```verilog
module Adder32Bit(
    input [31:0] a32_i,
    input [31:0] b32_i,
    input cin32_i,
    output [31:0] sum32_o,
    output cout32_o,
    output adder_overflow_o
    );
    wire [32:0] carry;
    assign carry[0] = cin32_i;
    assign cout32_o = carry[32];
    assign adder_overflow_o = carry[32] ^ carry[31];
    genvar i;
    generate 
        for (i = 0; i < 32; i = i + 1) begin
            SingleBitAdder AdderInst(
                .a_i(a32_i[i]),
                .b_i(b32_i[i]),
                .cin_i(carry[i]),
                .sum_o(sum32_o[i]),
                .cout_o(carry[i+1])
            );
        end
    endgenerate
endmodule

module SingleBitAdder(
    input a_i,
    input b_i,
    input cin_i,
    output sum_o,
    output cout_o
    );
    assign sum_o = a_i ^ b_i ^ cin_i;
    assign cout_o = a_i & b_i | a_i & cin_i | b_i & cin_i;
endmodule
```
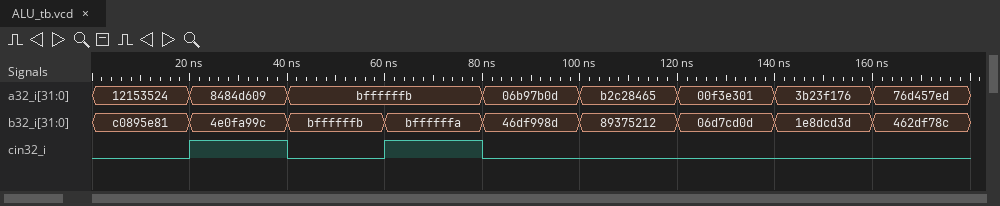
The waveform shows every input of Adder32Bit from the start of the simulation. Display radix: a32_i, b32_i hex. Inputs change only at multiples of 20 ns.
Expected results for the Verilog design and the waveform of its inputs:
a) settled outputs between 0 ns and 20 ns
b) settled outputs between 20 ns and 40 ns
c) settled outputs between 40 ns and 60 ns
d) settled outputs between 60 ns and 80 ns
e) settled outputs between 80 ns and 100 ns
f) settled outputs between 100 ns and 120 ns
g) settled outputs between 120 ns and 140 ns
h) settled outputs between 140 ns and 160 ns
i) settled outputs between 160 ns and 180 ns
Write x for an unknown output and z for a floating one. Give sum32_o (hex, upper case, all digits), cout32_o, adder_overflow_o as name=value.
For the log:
sum32_o=D29E93A5, cout32_o=0, adder_overflow_o=0
sum32_o=D2947FA6, cout32_o=0, adder_overflow_o=0
sum32_o=7FFFFFF6, cout32_o=1, adder_overflow_o=1
sum32_o=7FFFFFF6, cout32_o=1, adder_overflow_o=1
sum32_o=4D99149A, cout32_o=0, adder_overflow_o=0
sum32_o=3BF9D677, cout32_o=1, adder_overflow_o=1
sum32_o=07CBB00E, cout32_o=0, adder_overflow_o=0
sum32_o=59B1BEB3, cout32_o=0, adder_overflow_o=0
sum32_o=BD024F79, cout32_o=0, adder_overflow_o=1
